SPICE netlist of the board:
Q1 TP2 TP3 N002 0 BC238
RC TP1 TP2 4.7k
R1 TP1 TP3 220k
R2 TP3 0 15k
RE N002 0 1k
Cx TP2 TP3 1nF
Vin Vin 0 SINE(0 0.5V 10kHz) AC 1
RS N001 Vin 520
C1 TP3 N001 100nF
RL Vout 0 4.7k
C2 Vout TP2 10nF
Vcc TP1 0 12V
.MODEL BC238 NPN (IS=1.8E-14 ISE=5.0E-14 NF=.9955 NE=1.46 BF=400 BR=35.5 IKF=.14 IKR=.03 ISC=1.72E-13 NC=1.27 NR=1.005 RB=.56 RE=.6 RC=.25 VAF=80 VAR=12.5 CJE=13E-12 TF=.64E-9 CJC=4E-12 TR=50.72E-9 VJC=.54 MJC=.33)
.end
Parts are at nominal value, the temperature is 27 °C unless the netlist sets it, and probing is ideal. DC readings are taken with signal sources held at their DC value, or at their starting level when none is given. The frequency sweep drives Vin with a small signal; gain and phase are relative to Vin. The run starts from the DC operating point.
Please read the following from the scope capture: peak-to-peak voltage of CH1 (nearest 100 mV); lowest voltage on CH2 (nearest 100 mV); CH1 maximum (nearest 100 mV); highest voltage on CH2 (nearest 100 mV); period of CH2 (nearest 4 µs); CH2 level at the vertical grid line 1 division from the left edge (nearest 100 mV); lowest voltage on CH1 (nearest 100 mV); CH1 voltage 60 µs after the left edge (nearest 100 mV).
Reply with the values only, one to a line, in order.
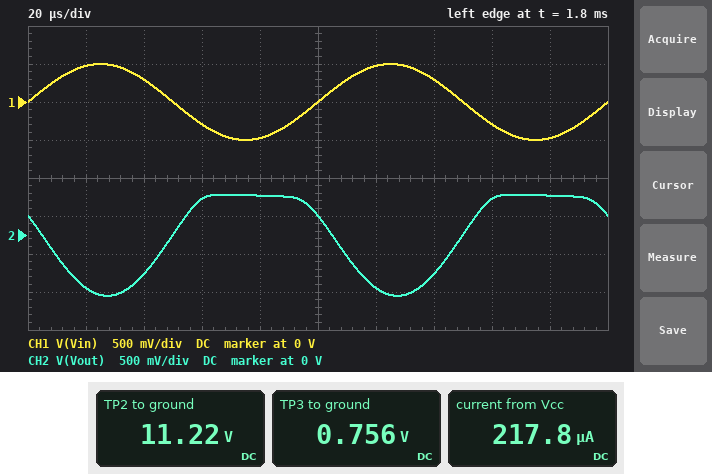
1.0 V
-800 mV
500 mV
500 mV
100 µs
-700 mV
-500 mV
-300 mV
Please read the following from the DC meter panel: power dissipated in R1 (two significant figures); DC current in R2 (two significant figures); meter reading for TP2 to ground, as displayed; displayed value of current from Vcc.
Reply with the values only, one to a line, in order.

570 µW
50 µA
11.22 V
217.8 µA
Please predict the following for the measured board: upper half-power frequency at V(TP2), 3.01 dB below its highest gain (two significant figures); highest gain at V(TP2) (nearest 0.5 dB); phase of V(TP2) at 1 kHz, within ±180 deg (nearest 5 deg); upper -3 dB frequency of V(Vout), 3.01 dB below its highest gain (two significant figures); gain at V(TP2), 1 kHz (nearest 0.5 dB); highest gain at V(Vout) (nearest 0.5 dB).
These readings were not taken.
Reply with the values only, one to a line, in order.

2.7 kHz
11.0 dB
170 deg
53 kHz
10.5 dB
5.0 dB
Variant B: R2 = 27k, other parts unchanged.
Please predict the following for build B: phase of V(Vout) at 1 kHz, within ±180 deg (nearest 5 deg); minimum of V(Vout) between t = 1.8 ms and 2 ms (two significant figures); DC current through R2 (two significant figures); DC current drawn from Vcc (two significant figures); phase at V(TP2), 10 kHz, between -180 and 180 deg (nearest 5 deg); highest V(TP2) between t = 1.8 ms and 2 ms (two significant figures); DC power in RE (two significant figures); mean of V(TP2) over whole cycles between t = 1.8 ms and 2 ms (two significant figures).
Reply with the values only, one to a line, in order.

-120 deg
-990 mV
47 µA
680 µA
155 deg
10 V
400 µW
9.0 V
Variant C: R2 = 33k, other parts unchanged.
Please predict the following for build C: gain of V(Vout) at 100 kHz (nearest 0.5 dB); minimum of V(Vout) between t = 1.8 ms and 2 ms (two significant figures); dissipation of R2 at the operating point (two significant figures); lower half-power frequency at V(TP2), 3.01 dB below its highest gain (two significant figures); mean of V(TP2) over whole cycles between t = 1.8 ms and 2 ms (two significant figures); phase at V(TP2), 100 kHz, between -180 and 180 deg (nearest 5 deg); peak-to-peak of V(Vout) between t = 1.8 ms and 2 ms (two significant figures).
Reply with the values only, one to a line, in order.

-0.5 dB
-1.0 V
66 µW
53 Hz
8.0 V
80 deg
2.0 V
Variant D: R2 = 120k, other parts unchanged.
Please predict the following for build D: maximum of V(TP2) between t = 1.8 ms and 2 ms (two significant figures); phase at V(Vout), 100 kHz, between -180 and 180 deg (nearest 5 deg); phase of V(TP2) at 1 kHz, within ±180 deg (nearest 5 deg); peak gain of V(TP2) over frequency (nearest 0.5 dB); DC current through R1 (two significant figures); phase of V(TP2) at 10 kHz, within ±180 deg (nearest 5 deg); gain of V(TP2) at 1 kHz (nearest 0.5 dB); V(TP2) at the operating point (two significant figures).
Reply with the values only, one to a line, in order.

4.2 V
80 deg
-145 deg
-5.0 dB
42 µA
165 deg
-6.0 dB
2.2 V
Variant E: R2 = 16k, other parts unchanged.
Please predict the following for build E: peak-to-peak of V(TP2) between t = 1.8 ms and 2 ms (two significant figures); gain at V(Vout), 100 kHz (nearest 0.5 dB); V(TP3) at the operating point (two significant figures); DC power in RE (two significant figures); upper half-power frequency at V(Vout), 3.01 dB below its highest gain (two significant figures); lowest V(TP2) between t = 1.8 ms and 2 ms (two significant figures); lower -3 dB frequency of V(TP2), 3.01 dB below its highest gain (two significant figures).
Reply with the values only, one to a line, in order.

1.6 V
-0.5 dB
800 mV
43 µW
52 kHz
9.9 V
93 Hz
